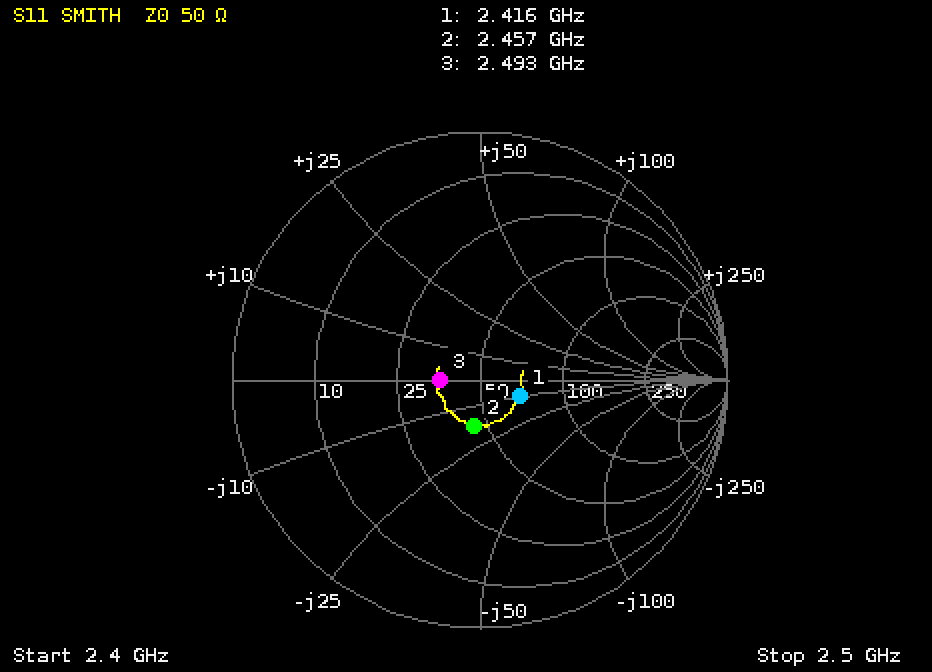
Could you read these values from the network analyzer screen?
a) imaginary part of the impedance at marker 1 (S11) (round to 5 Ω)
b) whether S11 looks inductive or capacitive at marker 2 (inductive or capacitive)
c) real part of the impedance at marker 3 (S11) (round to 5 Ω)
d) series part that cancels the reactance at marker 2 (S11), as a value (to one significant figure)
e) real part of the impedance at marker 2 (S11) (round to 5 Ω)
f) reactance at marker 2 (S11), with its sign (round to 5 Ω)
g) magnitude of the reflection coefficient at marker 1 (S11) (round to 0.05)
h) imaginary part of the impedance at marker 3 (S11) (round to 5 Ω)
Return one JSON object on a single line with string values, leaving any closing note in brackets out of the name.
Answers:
{"imaginary part of the impedance at marker 1 (S11)": "-10 Ω", "whether S11 looks inductive or capacitive at marker 2": "capacitive", "real part of the impedance at marker 3 (S11)": "35 Ω", "series part that cancels the reactance at marker 2 (S11), as a value": "1 nH", "real part of the impedance at marker 2 (S11)": "45 Ω", "reactance at marker 2 (S11), with its sign": "-15 Ω", "magnitude of the reflection coefficient at marker 1 (S11)": "0.15", "imaginary part of the impedance at marker 3 (S11)": "0 Ω"}
